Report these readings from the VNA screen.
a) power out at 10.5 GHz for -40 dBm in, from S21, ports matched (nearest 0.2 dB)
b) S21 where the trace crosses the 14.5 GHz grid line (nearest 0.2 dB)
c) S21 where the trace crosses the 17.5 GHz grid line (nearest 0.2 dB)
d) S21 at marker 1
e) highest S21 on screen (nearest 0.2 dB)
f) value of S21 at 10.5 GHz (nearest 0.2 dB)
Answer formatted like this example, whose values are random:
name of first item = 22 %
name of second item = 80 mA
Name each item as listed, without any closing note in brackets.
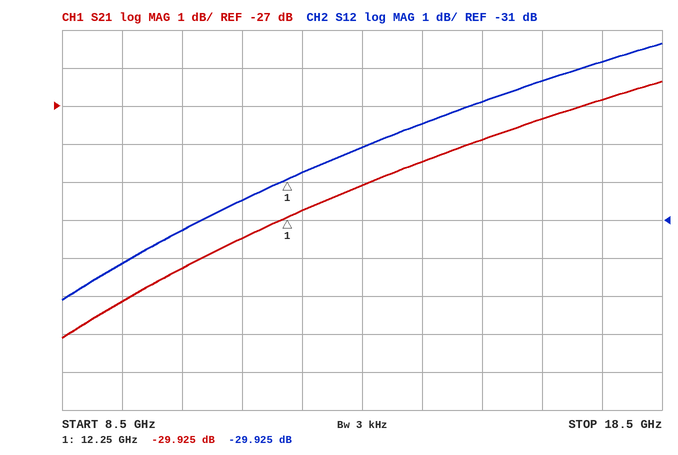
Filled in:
power out at 10.5 GHz for -40 dBm in, from S21, ports matched = -71.2 dBm
S21 where the trace crosses the 14.5 GHz grid line = -28.4 dB
S21 where the trace crosses the 17.5 GHz grid line = -26.8 dB
S21 at marker 1 = -29.925 dB
highest S21 on screen = -26.4 dB
value of S21 at 10.5 GHz = -31.2 dB
